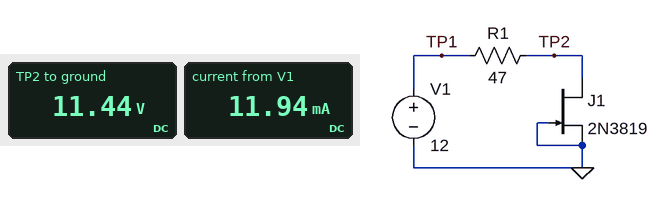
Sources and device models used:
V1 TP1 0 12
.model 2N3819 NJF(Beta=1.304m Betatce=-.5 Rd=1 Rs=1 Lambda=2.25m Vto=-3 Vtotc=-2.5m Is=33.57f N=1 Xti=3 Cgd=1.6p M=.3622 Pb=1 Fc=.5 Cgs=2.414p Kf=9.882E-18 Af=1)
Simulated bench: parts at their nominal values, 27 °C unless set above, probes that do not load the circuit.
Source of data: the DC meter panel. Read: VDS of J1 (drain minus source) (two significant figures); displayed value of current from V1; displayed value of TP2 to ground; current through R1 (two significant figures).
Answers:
11 V
11.94 mA
11.44 V
12 mA
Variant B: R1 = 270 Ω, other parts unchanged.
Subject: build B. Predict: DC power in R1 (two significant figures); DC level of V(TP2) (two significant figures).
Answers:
38 mW
8.8 V
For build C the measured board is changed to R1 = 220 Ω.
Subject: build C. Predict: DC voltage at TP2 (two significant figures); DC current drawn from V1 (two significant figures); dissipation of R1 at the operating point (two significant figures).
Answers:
9.4 V
12 mA
31 mW
